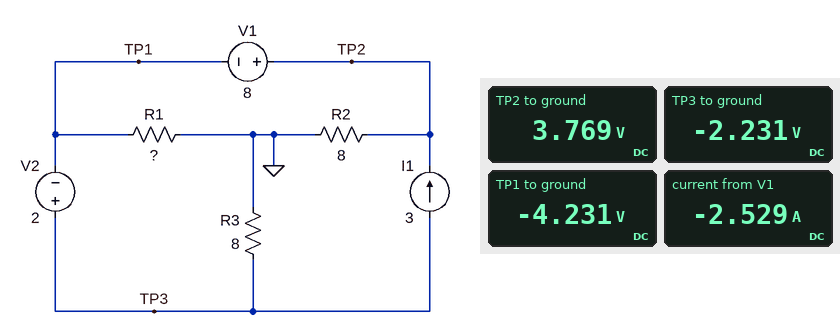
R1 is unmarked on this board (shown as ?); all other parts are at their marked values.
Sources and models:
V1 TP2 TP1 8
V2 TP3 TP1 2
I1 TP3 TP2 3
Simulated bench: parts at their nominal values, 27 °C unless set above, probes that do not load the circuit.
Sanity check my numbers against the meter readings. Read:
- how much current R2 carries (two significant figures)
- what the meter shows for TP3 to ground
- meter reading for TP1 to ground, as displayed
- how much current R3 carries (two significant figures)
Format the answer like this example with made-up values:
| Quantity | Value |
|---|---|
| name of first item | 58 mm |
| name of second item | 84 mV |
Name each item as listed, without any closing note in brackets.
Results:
| Quantity | Value |
|---|---|
| how much current R2 carries | 470 mA |
| what the meter shows for TP3 to ground | -2.231 V |
| meter reading for TP1 to ground, as displayed | -4.231 V |
| how much current R3 carries | 280 mA |
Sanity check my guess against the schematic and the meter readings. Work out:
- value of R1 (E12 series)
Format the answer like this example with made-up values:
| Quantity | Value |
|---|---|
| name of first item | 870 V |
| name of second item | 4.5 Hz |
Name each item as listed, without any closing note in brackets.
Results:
| Quantity | Value |
|---|---|
| value of R1 | 22 Ω |
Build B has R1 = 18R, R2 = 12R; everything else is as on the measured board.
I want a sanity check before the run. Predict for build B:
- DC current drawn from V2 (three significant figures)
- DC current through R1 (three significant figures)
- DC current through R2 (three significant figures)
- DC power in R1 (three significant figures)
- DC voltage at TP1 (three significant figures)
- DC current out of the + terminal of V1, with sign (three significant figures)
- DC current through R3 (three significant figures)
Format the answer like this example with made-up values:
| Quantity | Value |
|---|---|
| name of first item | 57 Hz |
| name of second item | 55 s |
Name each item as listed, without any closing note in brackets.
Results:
| Quantity | Value |
|---|---|
| DC current drawn from V2 | 2.82 A |
| DC current through R1 | 193 mA |
| DC current through R2 | 377 mA |
| DC power in R1 | 670 mW |
| DC voltage at TP1 | -3.47 V |
| DC current out of the + terminal of V1, with sign | -2.62 A |
| DC current through R3 | 184 mA |
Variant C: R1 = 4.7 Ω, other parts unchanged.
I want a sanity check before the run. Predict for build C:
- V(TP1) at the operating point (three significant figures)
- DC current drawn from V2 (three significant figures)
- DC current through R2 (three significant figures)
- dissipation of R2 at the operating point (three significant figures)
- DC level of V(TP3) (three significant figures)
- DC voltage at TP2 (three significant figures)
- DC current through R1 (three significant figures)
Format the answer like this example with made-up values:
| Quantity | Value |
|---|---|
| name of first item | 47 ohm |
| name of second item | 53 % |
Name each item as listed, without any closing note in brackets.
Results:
| Quantity | Value |
|---|---|
| V(TP1) at the operating point | -2.70 V |
| DC current drawn from V2 | 2.91 A |
| DC current through R2 | 662 mA |
| dissipation of R2 at the operating point | 3.51 W |
| DC level of V(TP3) | -701 mV |
| DC voltage at TP2 | 5.30 V |
| DC current through R1 | 575 mA |
